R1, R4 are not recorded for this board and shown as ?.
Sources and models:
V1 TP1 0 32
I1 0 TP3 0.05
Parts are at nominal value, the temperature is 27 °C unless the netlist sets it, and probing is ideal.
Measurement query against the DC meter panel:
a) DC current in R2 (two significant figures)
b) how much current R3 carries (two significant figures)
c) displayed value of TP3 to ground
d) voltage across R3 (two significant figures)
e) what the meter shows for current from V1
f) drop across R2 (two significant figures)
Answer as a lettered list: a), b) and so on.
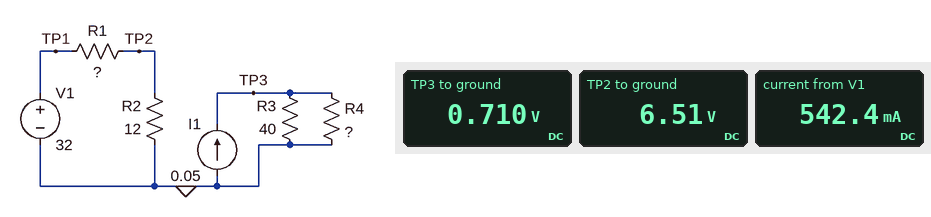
a) 540 mA
b) 18 mA
c) 0.710 V
d) 710 mV
e) 542.4 mA
f) 6.5 V
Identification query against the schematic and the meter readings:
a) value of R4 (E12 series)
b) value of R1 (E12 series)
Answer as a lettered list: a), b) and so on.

a) 22 Ω
b) 47 Ω
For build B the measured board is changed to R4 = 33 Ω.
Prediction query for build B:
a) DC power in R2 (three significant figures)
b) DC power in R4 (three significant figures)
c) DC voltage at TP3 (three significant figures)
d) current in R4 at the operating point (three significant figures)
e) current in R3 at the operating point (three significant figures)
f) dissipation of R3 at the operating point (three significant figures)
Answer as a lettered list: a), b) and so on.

a) 3.53 W
b) 24.8 mW
c) 904 mV
d) 27.4 mA
e) 22.6 mA
f) 20.4 mW
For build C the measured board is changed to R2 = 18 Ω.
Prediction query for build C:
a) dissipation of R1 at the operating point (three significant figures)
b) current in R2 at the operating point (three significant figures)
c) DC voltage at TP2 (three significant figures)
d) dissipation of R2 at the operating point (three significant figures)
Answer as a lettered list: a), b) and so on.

a) 11.4 W
b) 492 mA
c) 8.86 V
d) 4.36 W
